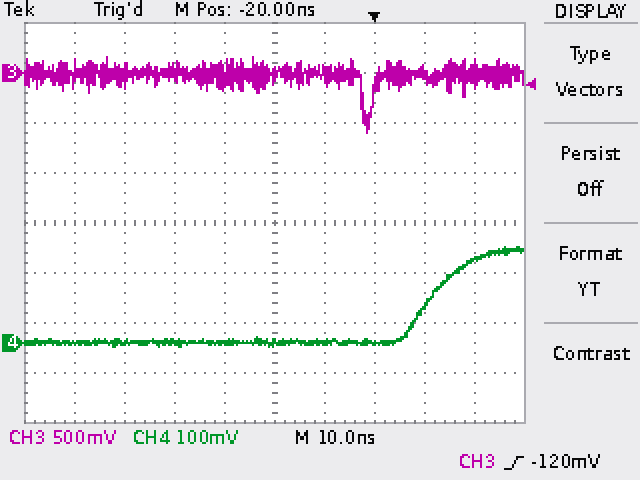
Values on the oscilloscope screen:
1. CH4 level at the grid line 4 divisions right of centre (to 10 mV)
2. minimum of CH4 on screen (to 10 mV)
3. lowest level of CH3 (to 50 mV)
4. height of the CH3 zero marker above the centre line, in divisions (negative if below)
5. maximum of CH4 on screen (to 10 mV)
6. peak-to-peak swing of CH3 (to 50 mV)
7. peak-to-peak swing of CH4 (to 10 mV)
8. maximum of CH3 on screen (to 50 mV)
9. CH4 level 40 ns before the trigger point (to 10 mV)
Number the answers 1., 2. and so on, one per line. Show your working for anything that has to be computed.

1. 170 mV
2. -10 mV
3. -600 mV
4. +3.0 div
5. 190 mV
6. 150 mV − (-600 mV) = 750 mV
7. 190 mV − (-10 mV) = 200 mV
8. 150 mV
9. 0 mV
